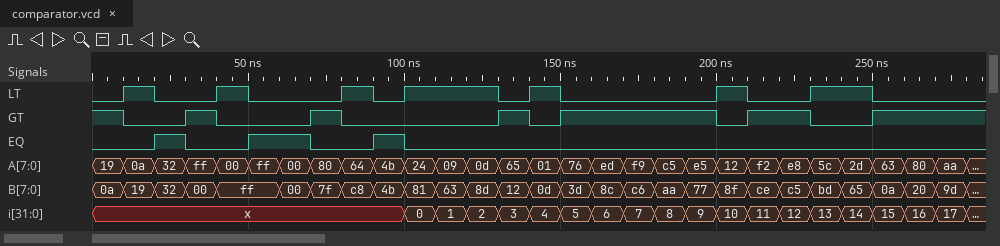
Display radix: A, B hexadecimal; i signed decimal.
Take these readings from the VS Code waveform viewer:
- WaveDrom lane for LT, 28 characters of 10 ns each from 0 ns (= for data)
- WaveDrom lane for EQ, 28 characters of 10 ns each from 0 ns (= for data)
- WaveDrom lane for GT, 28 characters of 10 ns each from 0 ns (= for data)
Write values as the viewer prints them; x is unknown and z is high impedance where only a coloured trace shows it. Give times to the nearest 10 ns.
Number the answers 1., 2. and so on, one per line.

1. {name: 'LT', wave: '010.10..101..010....10.1.0..'}
2. {name: 'EQ', wave: '0.10.1.0.10.................'}
3. {name: 'GT', wave: '10.10..10....101....01.0.1..'}
